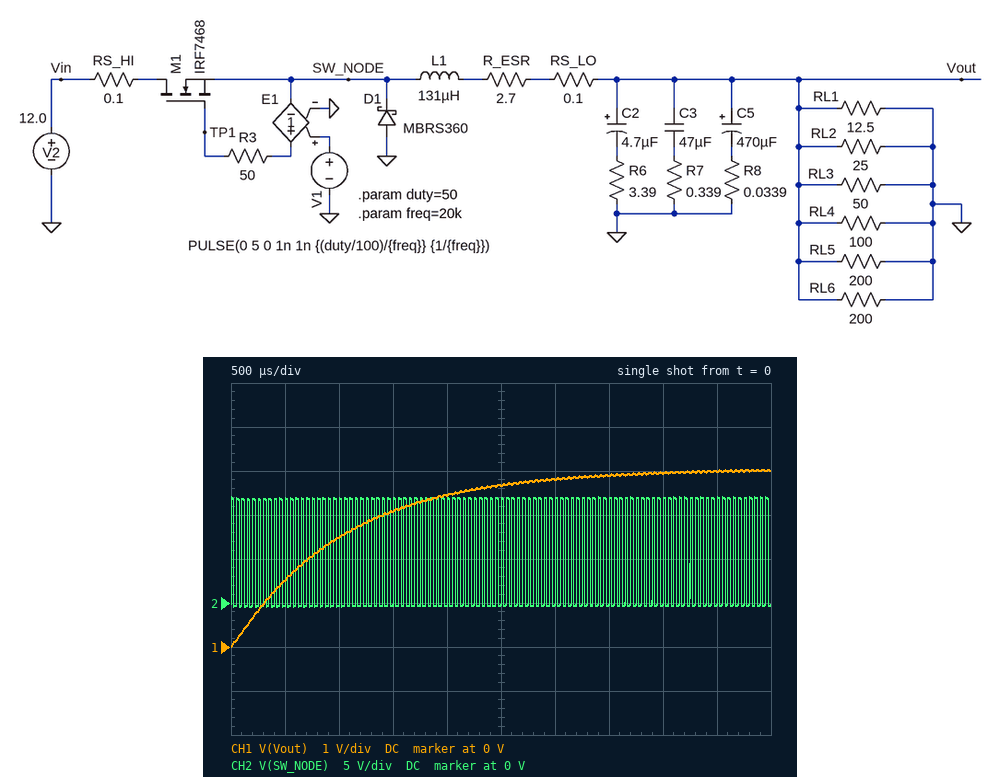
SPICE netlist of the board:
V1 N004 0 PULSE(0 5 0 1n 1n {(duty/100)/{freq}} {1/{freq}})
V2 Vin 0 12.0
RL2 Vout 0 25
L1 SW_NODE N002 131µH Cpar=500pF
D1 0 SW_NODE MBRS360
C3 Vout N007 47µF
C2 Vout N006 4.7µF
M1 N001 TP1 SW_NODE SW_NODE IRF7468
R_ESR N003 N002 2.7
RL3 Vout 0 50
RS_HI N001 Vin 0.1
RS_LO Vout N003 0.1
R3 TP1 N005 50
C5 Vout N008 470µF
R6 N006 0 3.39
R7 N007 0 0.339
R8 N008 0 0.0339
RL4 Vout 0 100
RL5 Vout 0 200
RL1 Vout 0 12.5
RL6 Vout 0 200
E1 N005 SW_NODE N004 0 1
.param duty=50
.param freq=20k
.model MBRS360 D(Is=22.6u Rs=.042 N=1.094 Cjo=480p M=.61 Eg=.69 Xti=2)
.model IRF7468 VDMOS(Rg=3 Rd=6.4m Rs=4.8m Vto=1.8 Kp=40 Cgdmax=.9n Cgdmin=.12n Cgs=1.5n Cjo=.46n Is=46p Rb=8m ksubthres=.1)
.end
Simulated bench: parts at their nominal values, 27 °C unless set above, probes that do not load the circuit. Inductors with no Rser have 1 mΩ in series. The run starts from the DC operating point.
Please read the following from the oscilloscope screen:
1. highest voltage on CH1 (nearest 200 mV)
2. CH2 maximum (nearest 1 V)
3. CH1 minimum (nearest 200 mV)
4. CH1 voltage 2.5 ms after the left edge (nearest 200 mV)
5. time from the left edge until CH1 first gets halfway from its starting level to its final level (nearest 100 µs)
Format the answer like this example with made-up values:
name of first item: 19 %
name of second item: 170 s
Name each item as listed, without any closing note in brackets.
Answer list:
highest voltage on CH1: 4.0 V
CH2 maximum: 12 V
CH1 minimum: 0 V
CH1 voltage 2.5 ms after the left edge: 3.6 V
time from the left edge until CH1 first gets halfway from its starting level to its final level: 700 µs
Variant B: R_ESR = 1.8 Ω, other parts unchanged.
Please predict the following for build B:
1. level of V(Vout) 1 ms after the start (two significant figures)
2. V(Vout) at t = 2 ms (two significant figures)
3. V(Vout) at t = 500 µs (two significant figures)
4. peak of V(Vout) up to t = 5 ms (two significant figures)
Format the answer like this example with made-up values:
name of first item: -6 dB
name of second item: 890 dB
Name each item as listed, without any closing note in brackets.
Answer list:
level of V(Vout) 1 ms after the start: 3.2 V
V(Vout) at t = 2 ms: 4.1 V
V(Vout) at t = 500 µs: 2.0 V
peak of V(Vout) up to t = 5 ms: 4.5 V
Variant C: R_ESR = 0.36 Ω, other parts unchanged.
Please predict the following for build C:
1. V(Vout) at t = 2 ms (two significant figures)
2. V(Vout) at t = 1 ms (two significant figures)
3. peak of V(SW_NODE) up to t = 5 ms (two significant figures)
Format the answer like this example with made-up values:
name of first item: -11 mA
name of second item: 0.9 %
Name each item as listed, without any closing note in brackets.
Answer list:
V(Vout) at t = 2 ms: 5.4 V
V(Vout) at t = 1 ms: 5.9 V
peak of V(SW_NODE) up to t = 5 ms: 12 V
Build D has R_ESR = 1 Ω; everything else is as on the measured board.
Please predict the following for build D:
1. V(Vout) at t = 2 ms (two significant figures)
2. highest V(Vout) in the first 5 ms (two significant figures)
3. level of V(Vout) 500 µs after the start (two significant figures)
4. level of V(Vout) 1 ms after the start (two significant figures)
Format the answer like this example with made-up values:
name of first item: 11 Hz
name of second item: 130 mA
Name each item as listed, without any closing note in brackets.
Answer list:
V(Vout) at t = 2 ms: 4.9 V
highest V(Vout) in the first 5 ms: 5.0 V
level of V(Vout) 500 µs after the start: 2.9 V
level of V(Vout) 1 ms after the start: 4.3 V
